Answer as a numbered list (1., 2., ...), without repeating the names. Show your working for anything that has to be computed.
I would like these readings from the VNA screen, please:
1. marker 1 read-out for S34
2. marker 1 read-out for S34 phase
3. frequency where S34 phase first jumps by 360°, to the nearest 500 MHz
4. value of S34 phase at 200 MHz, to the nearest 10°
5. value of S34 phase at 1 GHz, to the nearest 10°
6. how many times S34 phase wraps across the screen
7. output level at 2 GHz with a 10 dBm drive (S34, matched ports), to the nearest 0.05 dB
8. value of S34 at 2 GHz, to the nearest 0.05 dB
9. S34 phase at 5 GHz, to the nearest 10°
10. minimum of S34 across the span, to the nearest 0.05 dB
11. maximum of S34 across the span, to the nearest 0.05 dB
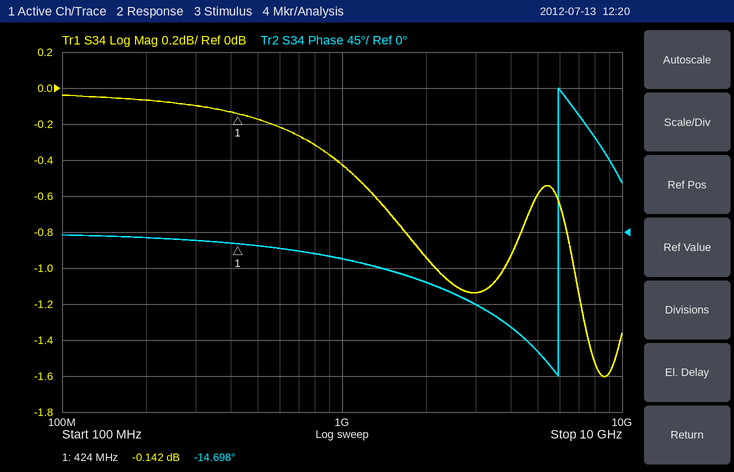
1. -0.142 dB
2. -14.698°
3. 6.0 GHz
4. -10°
5. -30°
6. 1
7. 10 dBm + (-0.95 dB) = 9.05 dBm
8. -0.95 dB
9. -150°
10. -1.60 dB
11. -0.05 dB
